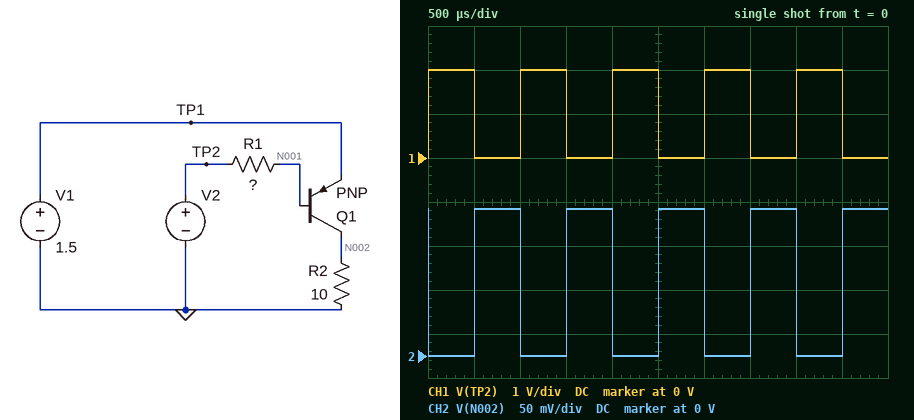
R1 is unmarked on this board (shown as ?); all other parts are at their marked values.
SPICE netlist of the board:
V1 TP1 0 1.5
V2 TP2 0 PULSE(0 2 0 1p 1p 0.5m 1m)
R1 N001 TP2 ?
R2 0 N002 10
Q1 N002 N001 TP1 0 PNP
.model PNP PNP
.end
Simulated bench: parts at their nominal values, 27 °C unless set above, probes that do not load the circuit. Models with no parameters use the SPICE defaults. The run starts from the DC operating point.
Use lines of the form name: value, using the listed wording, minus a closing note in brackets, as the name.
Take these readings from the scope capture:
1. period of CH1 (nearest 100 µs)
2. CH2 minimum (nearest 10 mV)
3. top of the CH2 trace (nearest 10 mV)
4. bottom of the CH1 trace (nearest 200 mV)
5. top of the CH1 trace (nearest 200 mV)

period of CH1: 1.0 ms
CH2 minimum: 0 V
top of the CH2 trace: 170 mV
bottom of the CH1 trace: 0 V
top of the CH1 trace: 2.0 V
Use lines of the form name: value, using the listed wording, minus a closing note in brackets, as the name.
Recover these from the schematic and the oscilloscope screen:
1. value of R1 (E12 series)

value of R1: 3.9 kΩ
